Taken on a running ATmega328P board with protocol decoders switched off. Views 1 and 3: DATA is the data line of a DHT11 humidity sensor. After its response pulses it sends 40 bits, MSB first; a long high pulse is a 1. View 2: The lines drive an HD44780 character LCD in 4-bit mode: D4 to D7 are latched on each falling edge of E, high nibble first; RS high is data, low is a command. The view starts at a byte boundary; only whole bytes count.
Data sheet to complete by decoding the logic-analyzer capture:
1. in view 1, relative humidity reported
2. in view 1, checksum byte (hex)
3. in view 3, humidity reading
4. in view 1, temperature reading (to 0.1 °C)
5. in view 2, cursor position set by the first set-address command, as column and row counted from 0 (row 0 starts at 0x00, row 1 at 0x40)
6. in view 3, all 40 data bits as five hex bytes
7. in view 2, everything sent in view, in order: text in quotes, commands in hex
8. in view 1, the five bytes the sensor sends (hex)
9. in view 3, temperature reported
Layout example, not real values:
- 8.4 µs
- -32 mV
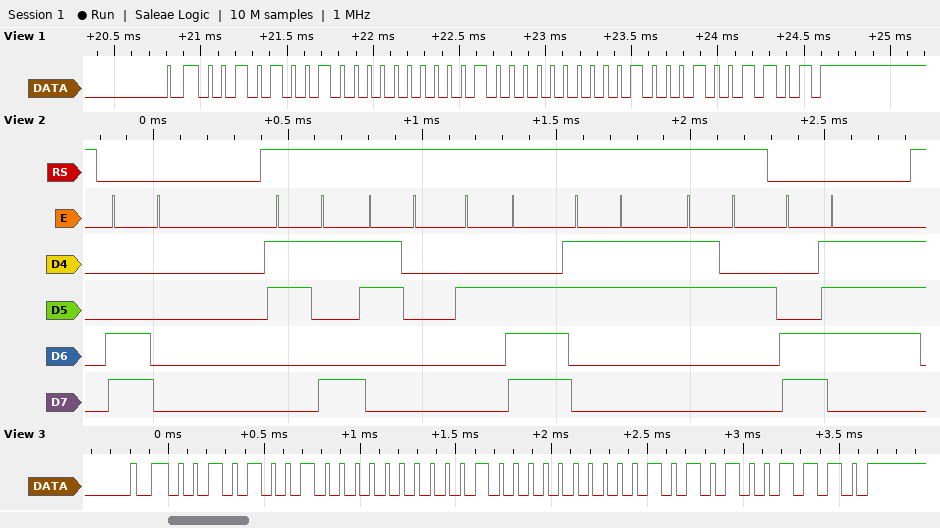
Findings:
- 41 %
- 0x4D
- 41 %
- 32.4 °C
- column 0, row 1
- 29 00 20 05 4E
- 0xC0 "90.32" 0xC7
- 29 00 20 04 4D
- 32.5 °C
